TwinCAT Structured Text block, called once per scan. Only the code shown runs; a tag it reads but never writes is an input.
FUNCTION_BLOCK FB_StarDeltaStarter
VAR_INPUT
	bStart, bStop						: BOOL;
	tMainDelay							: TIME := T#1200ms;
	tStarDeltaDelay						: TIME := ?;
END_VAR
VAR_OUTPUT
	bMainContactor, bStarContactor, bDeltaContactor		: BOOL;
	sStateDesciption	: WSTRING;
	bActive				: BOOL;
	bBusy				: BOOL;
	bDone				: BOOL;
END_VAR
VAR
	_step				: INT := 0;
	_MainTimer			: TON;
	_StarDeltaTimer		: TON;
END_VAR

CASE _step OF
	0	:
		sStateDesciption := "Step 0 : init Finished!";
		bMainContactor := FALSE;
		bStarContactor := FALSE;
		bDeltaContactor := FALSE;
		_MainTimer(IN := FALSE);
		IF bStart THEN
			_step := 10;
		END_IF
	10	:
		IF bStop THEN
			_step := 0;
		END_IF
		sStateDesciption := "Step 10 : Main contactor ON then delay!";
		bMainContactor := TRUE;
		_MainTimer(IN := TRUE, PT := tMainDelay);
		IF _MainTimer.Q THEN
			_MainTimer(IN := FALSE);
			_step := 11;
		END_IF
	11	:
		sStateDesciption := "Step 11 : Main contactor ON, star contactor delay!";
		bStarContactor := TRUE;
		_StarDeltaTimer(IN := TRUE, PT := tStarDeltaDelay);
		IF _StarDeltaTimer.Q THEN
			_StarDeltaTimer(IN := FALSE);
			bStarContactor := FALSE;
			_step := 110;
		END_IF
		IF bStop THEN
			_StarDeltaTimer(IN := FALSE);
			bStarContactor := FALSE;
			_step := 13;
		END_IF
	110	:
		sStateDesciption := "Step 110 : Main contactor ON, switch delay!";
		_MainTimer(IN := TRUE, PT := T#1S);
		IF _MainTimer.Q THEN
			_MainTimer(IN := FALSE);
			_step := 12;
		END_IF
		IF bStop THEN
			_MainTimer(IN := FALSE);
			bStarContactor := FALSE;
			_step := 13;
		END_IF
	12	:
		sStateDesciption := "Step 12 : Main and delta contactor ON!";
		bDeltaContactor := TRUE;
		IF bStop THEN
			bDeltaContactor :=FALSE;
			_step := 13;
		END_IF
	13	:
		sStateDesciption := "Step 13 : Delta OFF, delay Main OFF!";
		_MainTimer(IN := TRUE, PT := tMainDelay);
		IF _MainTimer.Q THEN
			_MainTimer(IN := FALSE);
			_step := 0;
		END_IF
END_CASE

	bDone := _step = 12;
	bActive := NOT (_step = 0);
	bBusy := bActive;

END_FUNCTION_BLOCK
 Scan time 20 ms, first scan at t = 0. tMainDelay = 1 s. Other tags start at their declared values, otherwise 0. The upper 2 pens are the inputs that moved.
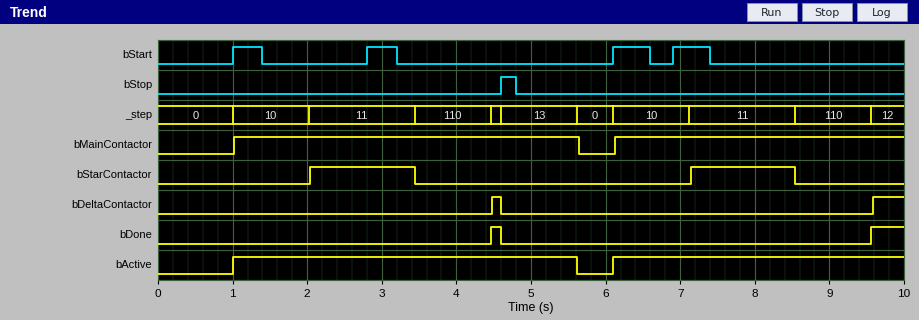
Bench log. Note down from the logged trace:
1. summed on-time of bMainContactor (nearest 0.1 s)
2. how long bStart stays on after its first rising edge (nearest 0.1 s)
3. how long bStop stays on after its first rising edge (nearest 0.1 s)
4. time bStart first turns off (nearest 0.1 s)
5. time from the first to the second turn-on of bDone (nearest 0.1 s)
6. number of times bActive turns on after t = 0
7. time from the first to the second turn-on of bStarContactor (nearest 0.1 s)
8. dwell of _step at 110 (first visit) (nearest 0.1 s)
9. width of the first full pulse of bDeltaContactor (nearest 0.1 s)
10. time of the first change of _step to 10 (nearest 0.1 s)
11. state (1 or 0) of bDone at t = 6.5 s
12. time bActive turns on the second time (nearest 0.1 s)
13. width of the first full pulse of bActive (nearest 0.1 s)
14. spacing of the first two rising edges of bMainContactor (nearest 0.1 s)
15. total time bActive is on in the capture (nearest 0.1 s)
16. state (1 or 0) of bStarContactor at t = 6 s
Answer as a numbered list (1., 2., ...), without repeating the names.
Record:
1. 8.5 s
2. 0.4 s
3. 0.2 s
4. 1.4 s
5. 5.1 s
6. 2
7. 5.1 s
8. 1.0 s
9. 0.1 s
10. 1.0 s
11. 0
12. 6.1 s
13. 4.6 s
14. 5.1 s
15. 8.5 s
16. 0
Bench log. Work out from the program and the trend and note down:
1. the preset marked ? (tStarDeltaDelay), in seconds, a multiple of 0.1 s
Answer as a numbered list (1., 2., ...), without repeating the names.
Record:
1. 1.4 s
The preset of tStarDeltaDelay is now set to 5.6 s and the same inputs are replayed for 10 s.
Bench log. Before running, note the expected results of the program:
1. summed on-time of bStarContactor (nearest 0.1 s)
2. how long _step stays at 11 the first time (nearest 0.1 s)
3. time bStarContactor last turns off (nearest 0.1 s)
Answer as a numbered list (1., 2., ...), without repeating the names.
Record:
1. 5.4 s
2. 2.6 s
3. 4.6 s
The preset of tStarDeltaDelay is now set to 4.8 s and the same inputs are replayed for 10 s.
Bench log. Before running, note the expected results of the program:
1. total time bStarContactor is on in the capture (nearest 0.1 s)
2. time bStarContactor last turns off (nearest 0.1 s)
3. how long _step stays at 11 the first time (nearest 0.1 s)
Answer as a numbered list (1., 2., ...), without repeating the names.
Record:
1. 5.4 s
2. 4.6 s
3. 2.6 s
